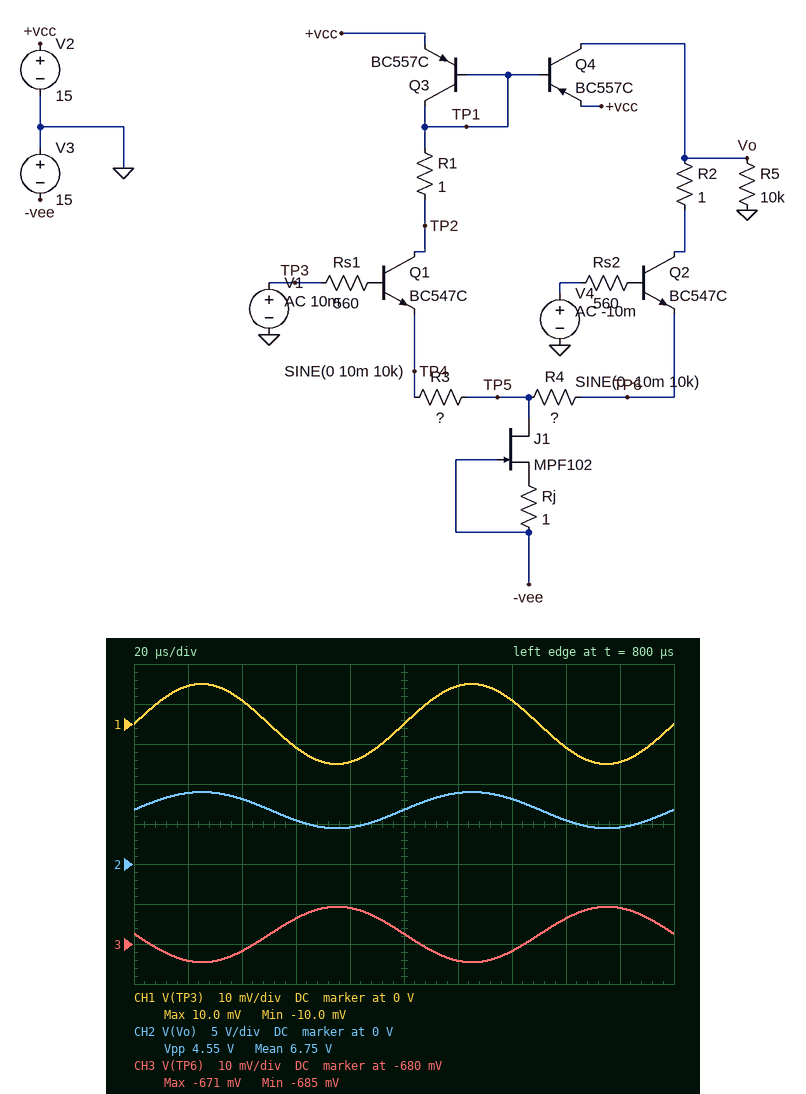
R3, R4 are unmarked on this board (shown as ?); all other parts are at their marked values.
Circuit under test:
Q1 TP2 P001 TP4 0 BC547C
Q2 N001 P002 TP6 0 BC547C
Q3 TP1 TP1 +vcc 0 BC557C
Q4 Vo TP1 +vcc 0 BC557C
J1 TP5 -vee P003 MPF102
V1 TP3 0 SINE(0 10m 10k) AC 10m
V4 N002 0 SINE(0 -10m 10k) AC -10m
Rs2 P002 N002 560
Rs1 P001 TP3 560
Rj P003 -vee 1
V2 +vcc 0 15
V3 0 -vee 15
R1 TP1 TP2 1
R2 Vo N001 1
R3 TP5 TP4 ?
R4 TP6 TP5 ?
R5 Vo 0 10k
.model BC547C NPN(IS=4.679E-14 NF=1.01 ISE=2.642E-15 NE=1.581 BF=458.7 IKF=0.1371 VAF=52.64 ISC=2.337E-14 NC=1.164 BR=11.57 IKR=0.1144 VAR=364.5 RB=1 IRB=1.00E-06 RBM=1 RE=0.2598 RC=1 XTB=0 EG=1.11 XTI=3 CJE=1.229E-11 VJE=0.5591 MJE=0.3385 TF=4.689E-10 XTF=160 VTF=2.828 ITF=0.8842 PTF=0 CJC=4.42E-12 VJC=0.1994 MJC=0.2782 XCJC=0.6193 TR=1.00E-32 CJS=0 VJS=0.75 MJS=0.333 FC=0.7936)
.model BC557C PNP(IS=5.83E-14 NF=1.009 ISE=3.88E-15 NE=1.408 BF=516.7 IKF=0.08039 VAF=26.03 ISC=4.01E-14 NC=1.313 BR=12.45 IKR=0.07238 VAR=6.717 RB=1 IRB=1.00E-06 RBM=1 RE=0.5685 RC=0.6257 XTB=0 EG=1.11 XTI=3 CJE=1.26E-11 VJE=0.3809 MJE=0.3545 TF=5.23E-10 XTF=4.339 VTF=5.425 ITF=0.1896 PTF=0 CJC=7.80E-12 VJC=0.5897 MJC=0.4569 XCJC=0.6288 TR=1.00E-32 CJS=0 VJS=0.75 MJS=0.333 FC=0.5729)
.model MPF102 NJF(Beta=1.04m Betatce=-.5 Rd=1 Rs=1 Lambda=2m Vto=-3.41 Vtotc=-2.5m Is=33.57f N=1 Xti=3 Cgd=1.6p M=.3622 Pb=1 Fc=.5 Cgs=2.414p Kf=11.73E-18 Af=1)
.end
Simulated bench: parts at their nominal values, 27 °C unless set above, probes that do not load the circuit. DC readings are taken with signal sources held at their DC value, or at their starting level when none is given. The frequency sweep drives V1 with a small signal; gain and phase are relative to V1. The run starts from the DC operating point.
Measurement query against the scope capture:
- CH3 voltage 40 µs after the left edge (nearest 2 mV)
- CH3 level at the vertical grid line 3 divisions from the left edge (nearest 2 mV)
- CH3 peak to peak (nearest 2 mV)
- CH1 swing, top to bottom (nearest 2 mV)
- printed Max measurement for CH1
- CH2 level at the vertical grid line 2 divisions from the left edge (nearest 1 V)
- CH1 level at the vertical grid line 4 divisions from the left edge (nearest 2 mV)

-682 mV
-674 mV
14 mV
20 mV
10.0 mV
8 V
-10 mV
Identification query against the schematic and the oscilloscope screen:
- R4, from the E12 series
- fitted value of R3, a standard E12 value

22 Ω
27 Ω
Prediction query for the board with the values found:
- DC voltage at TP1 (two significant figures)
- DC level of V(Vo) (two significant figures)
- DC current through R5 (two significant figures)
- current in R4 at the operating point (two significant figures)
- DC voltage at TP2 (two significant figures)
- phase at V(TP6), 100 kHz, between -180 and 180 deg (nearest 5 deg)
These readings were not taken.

14 V
6.8 V
680 µA
6.6 mA
14 V
20 deg
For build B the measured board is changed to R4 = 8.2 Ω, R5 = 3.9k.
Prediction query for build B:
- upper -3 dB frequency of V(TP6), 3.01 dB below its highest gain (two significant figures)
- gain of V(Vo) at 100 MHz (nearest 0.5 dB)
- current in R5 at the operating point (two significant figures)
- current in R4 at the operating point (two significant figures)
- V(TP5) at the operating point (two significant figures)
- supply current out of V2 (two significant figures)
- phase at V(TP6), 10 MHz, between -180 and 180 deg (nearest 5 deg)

120 MHz
-1.5 dB
160 µA
7.5 mA
-790 mV
12 mA
-5 deg
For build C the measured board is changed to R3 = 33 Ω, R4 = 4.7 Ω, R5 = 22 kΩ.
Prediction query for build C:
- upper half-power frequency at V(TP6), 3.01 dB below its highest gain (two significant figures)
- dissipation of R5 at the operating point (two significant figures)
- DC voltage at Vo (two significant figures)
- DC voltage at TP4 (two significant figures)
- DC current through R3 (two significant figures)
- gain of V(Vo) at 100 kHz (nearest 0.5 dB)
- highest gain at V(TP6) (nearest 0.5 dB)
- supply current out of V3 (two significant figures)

120 MHz
23 µW
-710 mV
-660 mV
4.7 mA
1.5 dB
0 dB
12 mA
